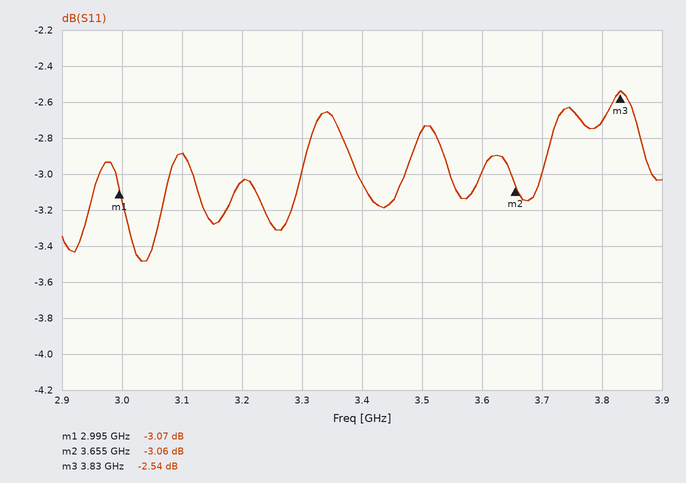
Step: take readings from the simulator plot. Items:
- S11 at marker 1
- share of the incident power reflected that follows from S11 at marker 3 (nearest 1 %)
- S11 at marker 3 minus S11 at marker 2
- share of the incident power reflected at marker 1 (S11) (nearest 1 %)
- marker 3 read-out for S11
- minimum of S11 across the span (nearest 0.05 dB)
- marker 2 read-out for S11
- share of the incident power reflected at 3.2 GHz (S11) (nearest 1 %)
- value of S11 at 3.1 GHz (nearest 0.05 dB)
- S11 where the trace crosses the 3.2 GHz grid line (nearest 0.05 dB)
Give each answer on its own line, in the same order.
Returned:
-3.07 dB
56 %
0.52 dB
49 %
-2.54 dB
-3.50 dB
-3.06 dB
50 %
-2.90 dB
-3.05 dB
